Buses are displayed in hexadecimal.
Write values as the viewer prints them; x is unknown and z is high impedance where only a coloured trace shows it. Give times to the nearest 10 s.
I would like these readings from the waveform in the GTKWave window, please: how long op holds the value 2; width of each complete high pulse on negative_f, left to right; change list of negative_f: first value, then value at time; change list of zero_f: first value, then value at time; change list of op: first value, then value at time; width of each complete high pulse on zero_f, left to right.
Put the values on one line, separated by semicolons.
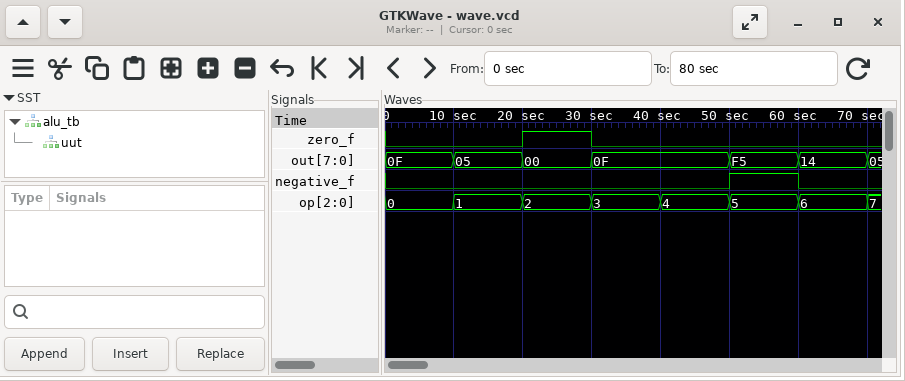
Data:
10 s; 10 s; 0, 1 at 50 s, 0 at 60 s; 0, 1 at 20 s, 0 at 30 s; 0, 1 at 10 s, 2 at 20 s, 3 at 30 s, 4 at 40 s, 5 at 50 s, 6 at 60 s, 7 at 70 s; 10 s
